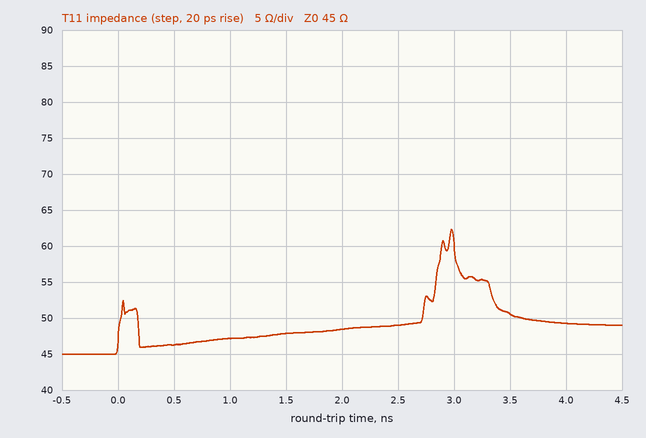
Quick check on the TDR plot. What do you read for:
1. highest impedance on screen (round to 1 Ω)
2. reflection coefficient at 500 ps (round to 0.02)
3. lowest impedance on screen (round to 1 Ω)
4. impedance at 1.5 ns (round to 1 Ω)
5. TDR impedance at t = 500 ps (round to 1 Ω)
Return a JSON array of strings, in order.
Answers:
["62 Ω", "+0.02", "45 Ω", "48 Ω", "46 Ω"]
